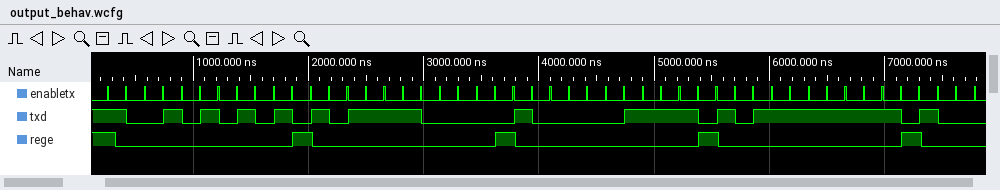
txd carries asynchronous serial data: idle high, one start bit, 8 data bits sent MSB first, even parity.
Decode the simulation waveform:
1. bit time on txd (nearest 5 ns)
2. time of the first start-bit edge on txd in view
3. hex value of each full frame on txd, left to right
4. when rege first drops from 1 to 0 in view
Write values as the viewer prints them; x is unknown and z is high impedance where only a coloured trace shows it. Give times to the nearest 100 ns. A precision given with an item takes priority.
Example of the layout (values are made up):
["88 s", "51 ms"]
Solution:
["160 ns", "400 ns", "55, F0, 0F, FF", "300 ns"]
